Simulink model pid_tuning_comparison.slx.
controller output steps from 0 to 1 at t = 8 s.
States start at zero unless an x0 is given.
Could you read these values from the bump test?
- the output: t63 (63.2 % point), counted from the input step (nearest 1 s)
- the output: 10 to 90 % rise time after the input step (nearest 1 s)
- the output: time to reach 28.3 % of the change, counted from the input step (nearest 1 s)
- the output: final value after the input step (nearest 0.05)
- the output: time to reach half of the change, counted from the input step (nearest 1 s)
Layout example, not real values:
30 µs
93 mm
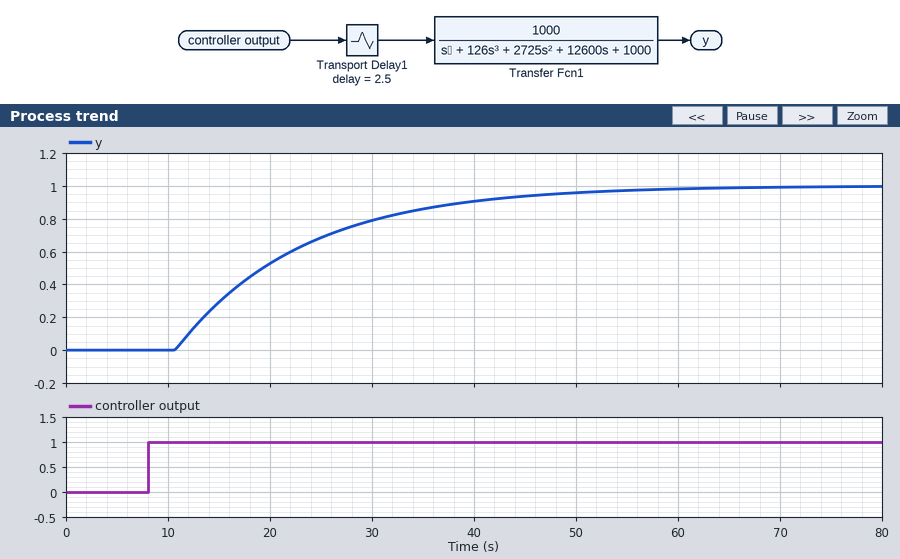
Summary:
15 s
27 s
7 s
1.00
11 s
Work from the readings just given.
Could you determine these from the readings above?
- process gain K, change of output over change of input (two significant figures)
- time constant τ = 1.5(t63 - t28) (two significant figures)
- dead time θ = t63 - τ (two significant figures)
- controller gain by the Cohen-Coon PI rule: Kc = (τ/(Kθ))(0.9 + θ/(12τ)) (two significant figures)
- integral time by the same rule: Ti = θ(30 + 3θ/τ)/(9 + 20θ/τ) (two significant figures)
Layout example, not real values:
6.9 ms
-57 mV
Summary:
1.0
12 s
3.0 s
3.7
6.6 s
